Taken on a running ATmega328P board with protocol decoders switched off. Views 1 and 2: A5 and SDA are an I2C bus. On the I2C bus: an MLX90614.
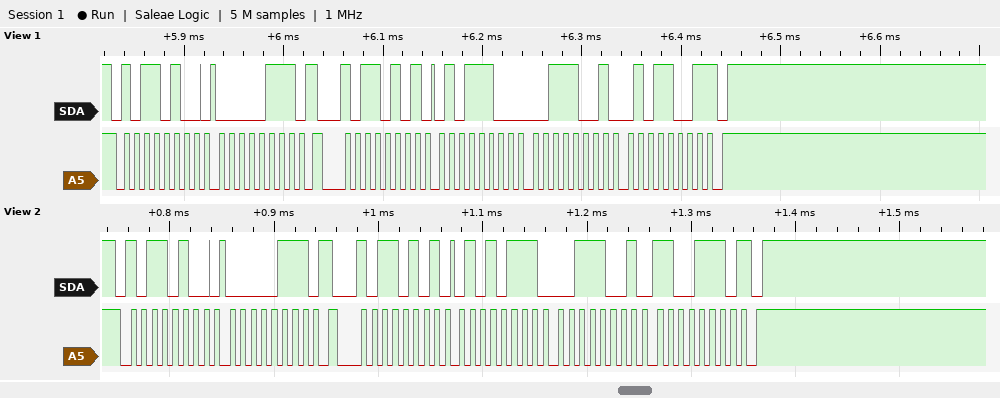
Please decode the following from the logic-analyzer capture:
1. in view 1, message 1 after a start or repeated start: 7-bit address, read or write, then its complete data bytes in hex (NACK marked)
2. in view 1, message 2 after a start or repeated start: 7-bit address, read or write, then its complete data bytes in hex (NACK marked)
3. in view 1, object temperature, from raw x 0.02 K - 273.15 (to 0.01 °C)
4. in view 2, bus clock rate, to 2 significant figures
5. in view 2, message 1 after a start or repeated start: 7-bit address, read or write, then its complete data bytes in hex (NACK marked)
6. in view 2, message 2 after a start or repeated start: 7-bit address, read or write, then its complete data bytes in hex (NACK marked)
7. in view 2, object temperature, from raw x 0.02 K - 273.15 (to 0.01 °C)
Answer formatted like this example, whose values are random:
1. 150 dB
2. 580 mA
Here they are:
1. 0x5A write: 07
2. 0x5A read: 5C 39 59 NACK
3. 20.53 °C
4. 100 kHz
5. 0x5A write: 07
6. 0x5A read: 57 39 CE NACK
7. 20.43 °C
